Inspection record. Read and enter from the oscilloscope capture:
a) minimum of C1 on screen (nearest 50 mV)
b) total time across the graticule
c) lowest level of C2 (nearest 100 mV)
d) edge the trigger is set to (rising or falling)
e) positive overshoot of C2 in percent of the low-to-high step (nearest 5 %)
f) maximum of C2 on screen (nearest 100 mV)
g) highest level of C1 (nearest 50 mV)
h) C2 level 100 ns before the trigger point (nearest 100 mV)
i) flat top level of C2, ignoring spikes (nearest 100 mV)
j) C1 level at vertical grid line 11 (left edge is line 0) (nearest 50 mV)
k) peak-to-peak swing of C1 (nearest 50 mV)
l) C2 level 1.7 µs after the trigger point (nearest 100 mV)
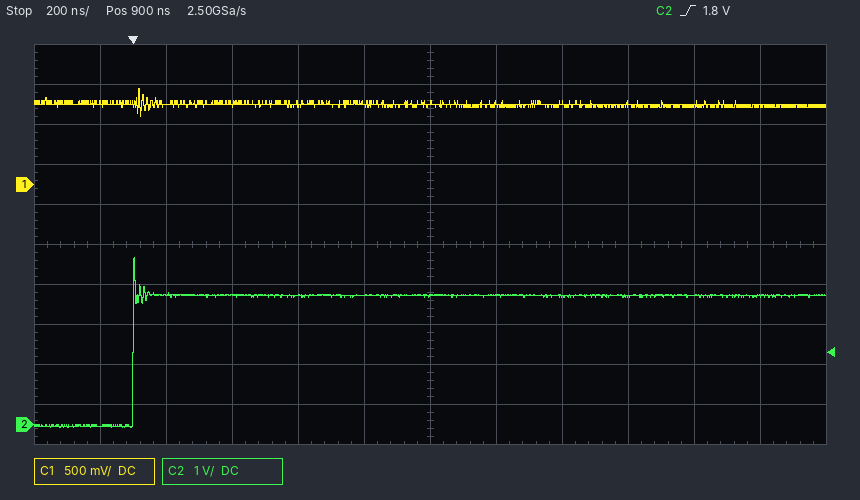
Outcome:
850 mV
2.4 µs
-100 mV
rising
30 %
4.2 V
1.20 V
0.0 V
3.2 V
1.00 V
350 mV
3.2 V
